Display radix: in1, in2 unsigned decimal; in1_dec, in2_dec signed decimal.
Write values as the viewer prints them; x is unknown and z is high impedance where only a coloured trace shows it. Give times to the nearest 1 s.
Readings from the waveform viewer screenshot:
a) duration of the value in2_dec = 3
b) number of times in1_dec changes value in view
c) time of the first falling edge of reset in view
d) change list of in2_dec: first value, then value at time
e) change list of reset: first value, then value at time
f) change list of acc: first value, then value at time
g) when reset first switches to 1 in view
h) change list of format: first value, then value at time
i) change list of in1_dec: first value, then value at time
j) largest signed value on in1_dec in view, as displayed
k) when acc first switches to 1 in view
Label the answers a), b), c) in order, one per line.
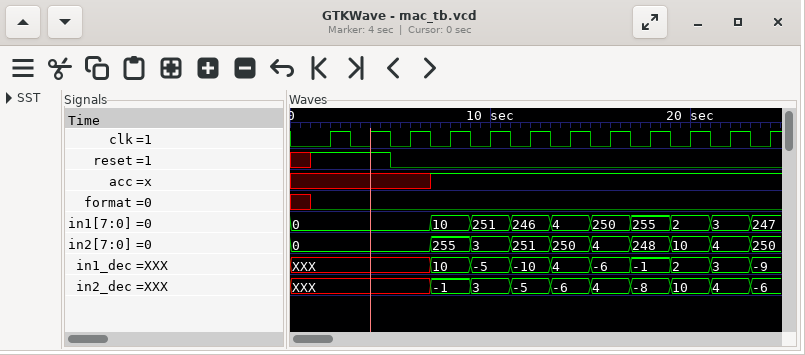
a) 2 s
b) 9
c) 5 s
d) XXX, -1 at 7 s, 3 at 9 s, -5 at 11 s, -6 at 13 s, 4 at 15 s, -8 at 17 s, 10 at 19 s, 4 at 21 s, -6 at 23 s
e) x, 1 at 1 s, 0 at 5 s
f) x, 1 at 7 s
g) 1 s
h) x, 0 at 1 s
i) XXX, 10 at 7 s, -5 at 9 s, -10 at 11 s, 4 at 13 s, -6 at 15 s, -1 at 17 s, 2 at 19 s, 3 at 21 s, -9 at 23 s
j) 10
k) 7 s
